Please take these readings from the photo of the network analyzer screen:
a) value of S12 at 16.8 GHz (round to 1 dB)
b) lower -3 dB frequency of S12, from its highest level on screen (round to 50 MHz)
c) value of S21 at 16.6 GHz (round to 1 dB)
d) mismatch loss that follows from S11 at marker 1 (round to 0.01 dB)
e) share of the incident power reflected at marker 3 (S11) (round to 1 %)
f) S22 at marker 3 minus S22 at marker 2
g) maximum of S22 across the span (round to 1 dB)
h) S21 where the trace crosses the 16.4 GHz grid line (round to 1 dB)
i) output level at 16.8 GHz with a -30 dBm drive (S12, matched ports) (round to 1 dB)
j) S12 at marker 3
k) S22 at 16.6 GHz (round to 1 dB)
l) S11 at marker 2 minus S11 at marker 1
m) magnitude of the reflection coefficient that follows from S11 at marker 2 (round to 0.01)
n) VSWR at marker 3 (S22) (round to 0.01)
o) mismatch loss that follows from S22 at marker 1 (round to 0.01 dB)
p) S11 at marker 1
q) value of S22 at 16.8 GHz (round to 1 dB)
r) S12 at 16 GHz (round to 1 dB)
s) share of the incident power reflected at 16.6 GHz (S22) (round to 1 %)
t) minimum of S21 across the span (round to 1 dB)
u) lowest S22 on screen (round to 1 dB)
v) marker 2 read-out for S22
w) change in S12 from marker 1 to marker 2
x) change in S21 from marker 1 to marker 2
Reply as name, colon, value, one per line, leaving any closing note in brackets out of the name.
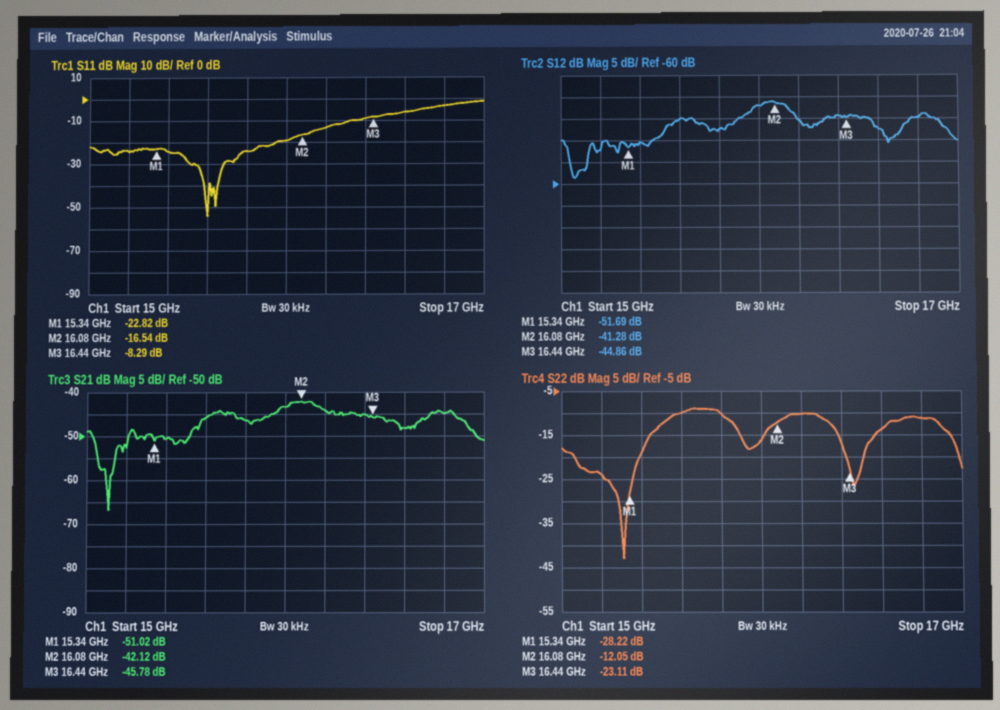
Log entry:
value of S12 at 16.8 GHz: -45 dB
lower -3 dB frequency of S12, from its highest level on screen: 15.95 GHz
value of S21 at 16.6 GHz: -48 dB
mismatch loss that follows from S11 at marker 1: 0.02 dB
share of the incident power reflected at marker 3 (S11): 15 %
S22 at marker 3 minus S22 at marker 2: -11.06 dB
maximum of S22 across the span: -9 dB
S21 where the trace crosses the 16.4 GHz grid line: -45 dB
output level at 16.8 GHz with a -30 dBm drive (S12, matched ports): -75 dBm
S12 at marker 3: -44.86 dB
S22 at 16.6 GHz: -14 dB
S11 at marker 2 minus S11 at marker 1: 6.28 dB
magnitude of the reflection coefficient that follows from S11 at marker 2: 0.15
VSWR at marker 3 (S22): 1.15
mismatch loss that follows from S22 at marker 1: 0.01 dB
S11 at marker 1: -22.82 dB
value of S22 at 16.8 GHz: -11 dB
S12 at 16 GHz: -42 dB
share of the incident power reflected at 16.6 GHz (S22): 4 %
minimum of S21 across the span: -67 dB
lowest S22 on screen: -43 dB
marker 2 read-out for S22: -12.05 dB
change in S12 from marker 1 to marker 2: 10.41 dB
change in S21 from marker 1 to marker 2: 8.90 dB
